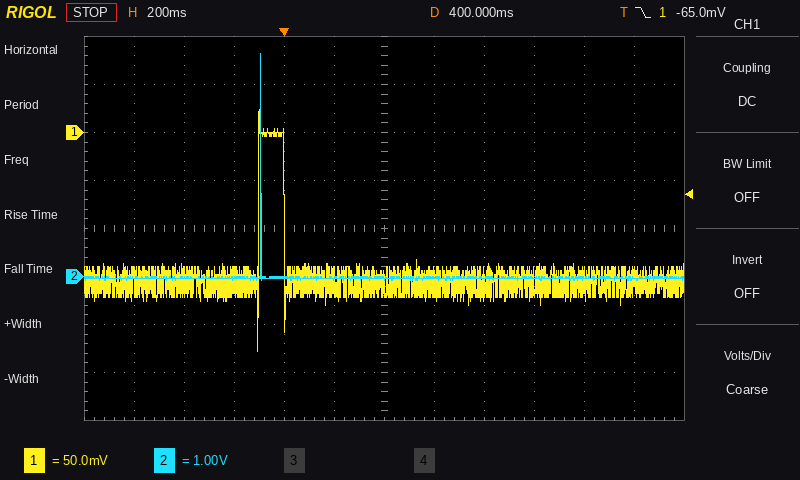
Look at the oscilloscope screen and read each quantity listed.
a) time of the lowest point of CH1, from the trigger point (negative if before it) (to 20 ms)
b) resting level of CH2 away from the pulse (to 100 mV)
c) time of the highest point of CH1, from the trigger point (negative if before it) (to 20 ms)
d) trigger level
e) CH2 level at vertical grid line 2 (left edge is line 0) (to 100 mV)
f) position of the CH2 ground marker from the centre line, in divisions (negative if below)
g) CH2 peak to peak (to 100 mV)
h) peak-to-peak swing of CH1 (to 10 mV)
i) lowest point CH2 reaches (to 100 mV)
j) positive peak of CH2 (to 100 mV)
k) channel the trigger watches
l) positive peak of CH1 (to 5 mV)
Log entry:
-100 ms
0.0 V
-100 ms
-65.0 mV
0.0 V
-1.0 div
4.7 V
250 mV
-100 mV
4.6 V
CH1
25 mV
